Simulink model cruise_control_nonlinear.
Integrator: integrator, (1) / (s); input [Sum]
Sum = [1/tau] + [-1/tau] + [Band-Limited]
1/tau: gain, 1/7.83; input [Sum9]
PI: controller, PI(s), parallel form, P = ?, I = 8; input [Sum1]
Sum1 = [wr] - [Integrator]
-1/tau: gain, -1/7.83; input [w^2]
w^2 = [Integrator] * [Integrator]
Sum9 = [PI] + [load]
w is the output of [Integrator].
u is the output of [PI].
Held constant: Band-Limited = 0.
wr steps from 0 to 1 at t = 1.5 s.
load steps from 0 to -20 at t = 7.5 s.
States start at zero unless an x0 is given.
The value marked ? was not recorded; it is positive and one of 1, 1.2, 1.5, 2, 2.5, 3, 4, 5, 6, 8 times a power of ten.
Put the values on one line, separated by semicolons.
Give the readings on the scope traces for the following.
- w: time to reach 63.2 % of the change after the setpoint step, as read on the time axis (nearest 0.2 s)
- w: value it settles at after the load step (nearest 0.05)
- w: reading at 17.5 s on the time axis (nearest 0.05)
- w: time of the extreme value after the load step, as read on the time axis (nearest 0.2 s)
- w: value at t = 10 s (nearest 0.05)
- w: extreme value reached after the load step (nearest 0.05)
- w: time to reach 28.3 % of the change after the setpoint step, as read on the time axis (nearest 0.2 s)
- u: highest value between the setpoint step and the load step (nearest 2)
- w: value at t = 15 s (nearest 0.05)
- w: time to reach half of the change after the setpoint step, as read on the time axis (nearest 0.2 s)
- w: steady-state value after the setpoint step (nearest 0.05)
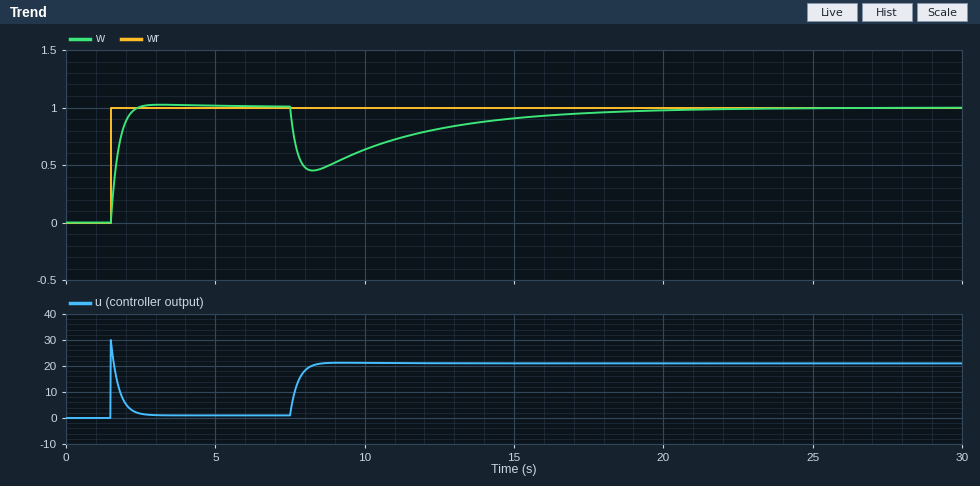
1.8 s; 1.00; 0.95; 8.2 s; 0.65; 0.45; 1.6 s; 30; 0.90; 1.6 s; 1.00
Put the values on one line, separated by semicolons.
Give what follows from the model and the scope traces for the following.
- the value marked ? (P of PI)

30
